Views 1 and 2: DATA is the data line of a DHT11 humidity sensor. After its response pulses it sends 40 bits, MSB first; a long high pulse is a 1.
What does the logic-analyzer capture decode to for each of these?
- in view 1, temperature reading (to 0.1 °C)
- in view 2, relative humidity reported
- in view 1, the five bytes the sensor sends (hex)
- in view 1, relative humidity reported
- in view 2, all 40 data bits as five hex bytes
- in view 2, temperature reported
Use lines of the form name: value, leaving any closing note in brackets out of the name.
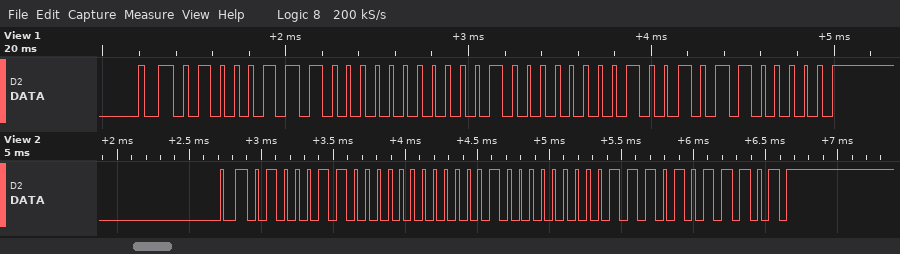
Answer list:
in view 1, temperature reading: 16.9 °C
in view 2, relative humidity reported: 70 %
in view 1, the five bytes the sensor sends: 47 00 10 09 60
in view 1, relative humidity reported: 71 %
in view 2, all 40 data bits as five hex bytes: 46 00 10 07 5D
in view 2, temperature reported: 16.7 °C
